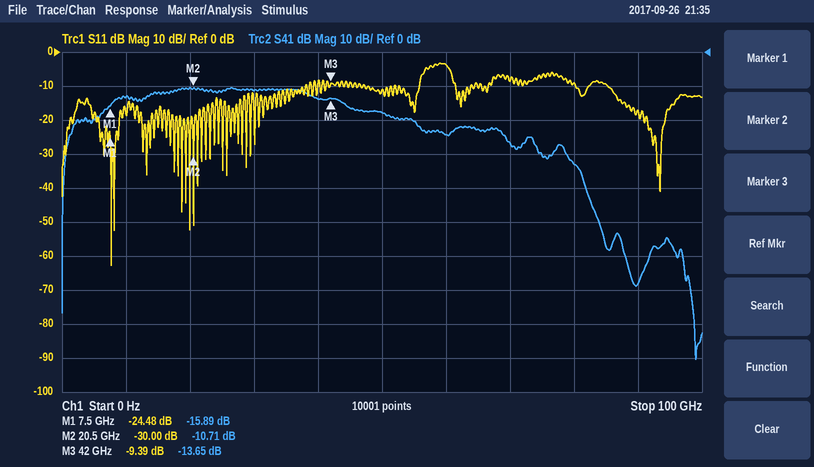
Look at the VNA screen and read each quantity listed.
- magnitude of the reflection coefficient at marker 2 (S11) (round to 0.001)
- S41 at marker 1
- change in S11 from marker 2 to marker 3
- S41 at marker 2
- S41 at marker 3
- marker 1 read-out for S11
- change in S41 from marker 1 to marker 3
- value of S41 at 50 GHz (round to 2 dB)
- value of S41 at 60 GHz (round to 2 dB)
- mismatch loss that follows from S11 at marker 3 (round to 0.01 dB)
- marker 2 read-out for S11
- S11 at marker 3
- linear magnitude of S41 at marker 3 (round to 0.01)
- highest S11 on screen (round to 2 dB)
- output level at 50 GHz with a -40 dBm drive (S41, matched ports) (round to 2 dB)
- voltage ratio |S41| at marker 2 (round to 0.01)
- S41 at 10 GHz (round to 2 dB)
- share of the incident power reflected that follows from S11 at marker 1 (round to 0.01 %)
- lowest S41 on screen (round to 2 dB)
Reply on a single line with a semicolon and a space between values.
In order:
0.032; -15.89 dB; 20.61 dB; -10.71 dB; -13.65 dB; -24.48 dB; 2.24 dB; -18 dB; -24 dB; 0.53 dB; -30.00 dB; -9.39 dB; 0.21; -4 dB; -58 dBm; 0.29; -14 dB; 0.36 %; -90 dB
